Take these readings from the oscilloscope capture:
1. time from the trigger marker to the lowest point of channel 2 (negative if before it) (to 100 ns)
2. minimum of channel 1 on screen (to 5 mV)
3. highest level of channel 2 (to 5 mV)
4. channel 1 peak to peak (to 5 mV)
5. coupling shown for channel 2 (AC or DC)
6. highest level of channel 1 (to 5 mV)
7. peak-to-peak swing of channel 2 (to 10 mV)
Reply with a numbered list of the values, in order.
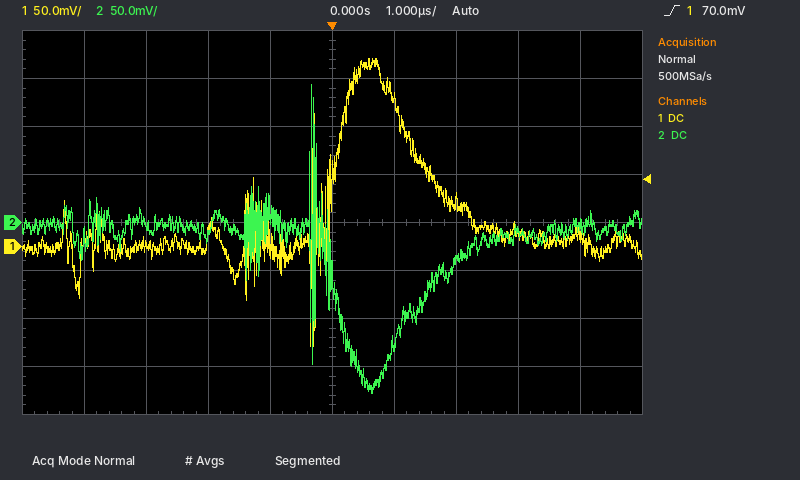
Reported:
1. +600 ns
2. -105 mV
3. 145 mV
4. 300 mV
5. DC
6. 195 mV
7. 320 mV
